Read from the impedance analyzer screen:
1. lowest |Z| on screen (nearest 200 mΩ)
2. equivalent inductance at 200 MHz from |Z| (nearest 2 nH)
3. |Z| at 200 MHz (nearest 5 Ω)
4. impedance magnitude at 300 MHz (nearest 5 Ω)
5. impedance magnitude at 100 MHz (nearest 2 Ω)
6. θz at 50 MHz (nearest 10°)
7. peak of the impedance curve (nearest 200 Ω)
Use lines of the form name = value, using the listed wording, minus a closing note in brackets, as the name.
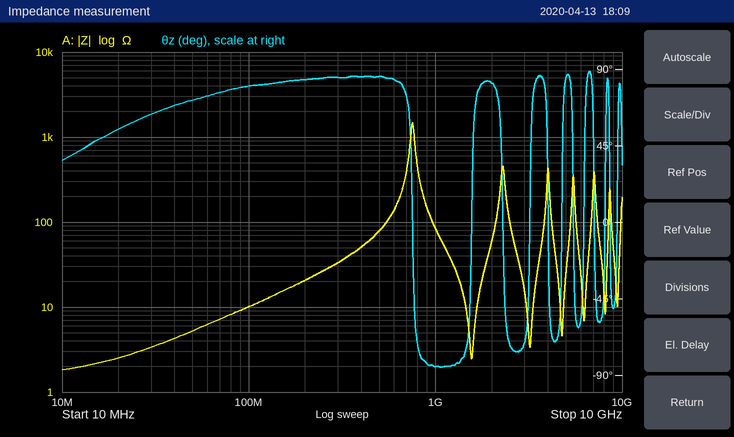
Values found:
lowest |Z| on screen = 1.8 Ω
equivalent inductance at 200 MHz from |Z| = 16 nH
|Z| at 200 MHz = 20 Ω
impedance magnitude at 300 MHz = 35 Ω
impedance magnitude at 100 MHz = 10 Ω
θz at 50 MHz = 70°
peak of the impedance curve = 1.4 kΩ
